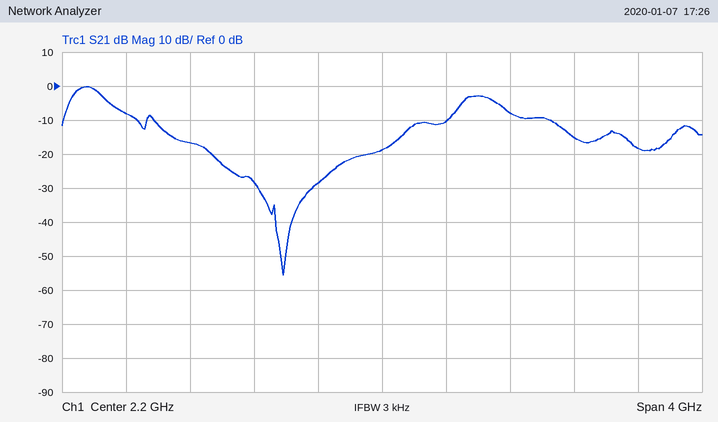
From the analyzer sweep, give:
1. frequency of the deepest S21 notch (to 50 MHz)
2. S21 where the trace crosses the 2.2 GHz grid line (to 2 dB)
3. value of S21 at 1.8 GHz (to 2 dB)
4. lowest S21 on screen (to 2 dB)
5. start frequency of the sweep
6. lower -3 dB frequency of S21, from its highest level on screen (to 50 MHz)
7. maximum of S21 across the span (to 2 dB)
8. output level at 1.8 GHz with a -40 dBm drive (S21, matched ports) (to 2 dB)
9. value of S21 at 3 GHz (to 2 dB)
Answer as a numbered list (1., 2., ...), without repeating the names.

1. 1.60 GHz
2. -18 dB
3. -28 dB
4. -56 dB
5. 200 MHz
6. 250 MHz
7. 0 dB
8. -68 dBm
9. -8 dB
